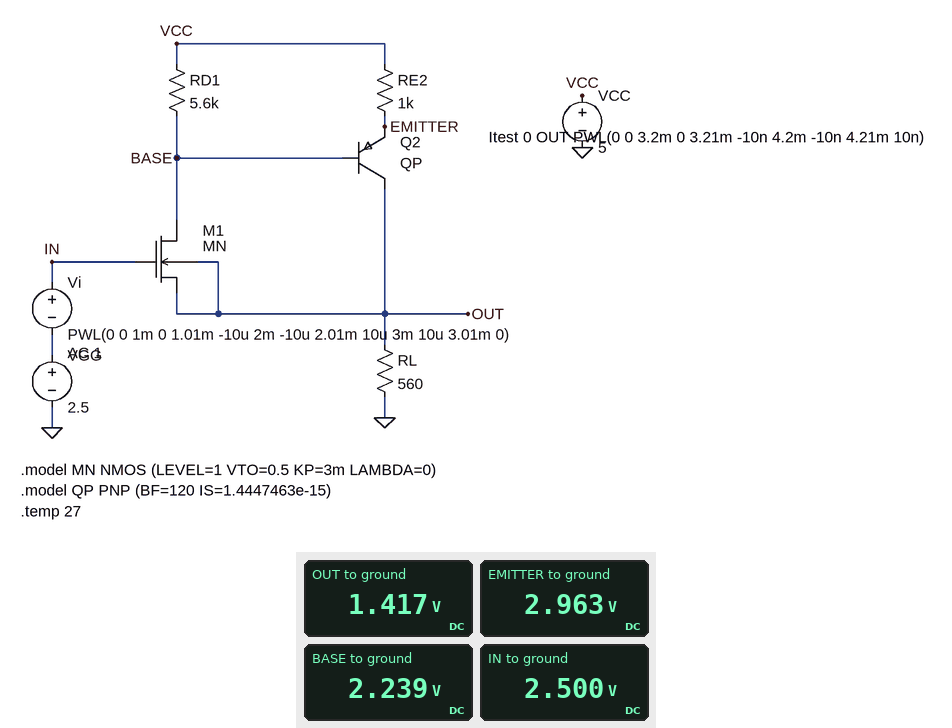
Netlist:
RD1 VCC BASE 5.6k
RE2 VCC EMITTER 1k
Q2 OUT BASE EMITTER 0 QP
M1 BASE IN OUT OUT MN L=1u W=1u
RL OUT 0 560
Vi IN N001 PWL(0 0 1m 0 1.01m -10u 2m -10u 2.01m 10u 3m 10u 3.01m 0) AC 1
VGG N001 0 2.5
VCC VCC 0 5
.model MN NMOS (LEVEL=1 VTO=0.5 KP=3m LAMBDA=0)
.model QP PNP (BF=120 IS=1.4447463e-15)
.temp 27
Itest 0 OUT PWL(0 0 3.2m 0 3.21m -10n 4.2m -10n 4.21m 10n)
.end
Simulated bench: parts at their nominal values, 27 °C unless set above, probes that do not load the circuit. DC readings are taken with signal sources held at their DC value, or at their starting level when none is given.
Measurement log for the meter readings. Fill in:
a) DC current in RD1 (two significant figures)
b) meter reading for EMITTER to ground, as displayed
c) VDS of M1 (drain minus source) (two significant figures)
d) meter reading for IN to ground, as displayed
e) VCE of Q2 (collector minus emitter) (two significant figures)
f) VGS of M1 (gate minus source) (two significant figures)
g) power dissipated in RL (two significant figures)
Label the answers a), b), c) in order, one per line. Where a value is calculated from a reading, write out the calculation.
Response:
a) (5 V - 2.239 V) / 5.6 kΩ = 490 µA
b) 2.963 V
c) 2.239 V - 1.417 V = 820 mV
d) 2.500 V
e) 1.417 V - 2.963 V = -1.5 V
f) 2.5 V - 1.417 V = 1.1 V
g) (1.417 V)^2 / 560 Ω = 3.6 mW
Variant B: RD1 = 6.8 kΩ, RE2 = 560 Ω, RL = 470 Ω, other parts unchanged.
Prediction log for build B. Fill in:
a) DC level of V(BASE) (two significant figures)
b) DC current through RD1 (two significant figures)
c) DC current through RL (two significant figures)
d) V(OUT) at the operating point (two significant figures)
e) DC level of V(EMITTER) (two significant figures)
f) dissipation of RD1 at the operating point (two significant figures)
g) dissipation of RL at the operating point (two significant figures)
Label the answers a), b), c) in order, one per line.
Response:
a) 2.7 V
b) 340 µA
c) 3.2 mA
d) 1.5 V
e) 3.4 V
f) 800 µW
g) 4.8 mW
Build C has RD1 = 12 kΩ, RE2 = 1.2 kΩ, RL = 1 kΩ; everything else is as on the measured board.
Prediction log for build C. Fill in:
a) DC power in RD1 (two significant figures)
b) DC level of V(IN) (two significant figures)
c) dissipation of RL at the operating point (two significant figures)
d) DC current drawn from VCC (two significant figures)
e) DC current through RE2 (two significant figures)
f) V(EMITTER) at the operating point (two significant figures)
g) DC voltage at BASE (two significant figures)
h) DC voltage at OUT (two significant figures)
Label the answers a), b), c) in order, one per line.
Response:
a) 490 µW
b) 2.5 V
c) 2.6 mW
d) 1.6 mA
e) 1.4 mA
f) 3.3 V
g) 2.6 V
h) 1.6 V
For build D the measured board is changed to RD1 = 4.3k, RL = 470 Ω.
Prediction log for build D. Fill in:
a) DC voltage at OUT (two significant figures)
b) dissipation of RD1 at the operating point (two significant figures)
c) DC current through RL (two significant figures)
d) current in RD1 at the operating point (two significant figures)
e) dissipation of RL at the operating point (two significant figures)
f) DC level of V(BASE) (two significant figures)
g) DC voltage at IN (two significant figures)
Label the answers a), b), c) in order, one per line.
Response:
a) 1.3 V
b) 1.9 mW
c) 2.8 mA
d) 670 µA
e) 3.7 mW
f) 2.1 V
g) 2.5 V
